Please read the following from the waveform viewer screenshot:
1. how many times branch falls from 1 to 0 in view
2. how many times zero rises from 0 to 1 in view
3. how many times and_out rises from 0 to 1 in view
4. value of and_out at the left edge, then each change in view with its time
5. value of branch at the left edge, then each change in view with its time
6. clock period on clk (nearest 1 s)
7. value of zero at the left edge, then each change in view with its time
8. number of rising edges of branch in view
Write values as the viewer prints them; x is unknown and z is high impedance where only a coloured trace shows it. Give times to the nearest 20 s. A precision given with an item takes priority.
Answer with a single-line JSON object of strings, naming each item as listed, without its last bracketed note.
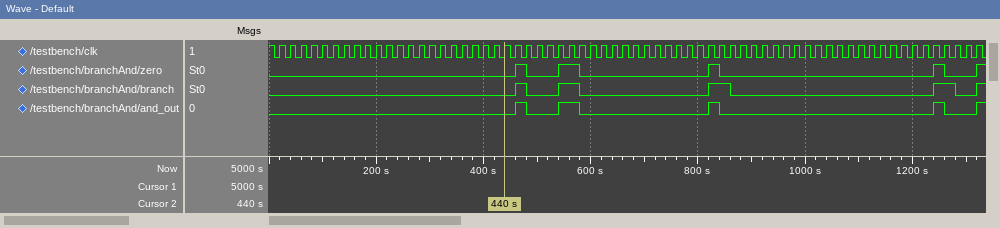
{"how many times branch falls from 1 to 0 in view": "4", "how many times zero rises from 0 to 1 in view": "5", "how many times and_out rises from 0 to 1 in view": "5", "value of and_out at the left edge, then each change in view with its time": "0, 1 at 460 s, 0 at 480 s, 1 at 540 s, 0 at 580 s, 1 at 820 s, 0 at 840 s, 1 at 1240 s, 0 at 1260 s, 1 at 1320 s", "value of branch at the left edge, then each change in view with its time": "0, 1 at 460 s, 0 at 480 s, 1 at 540 s, 0 at 580 s, 1 at 820 s, 0 at 860 s, 1 at 1240 s, 0 at 1280 s, 1 at 1320 s", "clock period on clk": "20 s", "value of zero at the left edge, then each change in view with its time": "0, 1 at 460 s, 0 at 480 s, 1 at 540 s, 0 at 580 s, 1 at 820 s, 0 at 840 s, 1 at 1240 s, 0 at 1260 s, 1 at 1320 s", "number of rising edges of branch in view": "5"}
